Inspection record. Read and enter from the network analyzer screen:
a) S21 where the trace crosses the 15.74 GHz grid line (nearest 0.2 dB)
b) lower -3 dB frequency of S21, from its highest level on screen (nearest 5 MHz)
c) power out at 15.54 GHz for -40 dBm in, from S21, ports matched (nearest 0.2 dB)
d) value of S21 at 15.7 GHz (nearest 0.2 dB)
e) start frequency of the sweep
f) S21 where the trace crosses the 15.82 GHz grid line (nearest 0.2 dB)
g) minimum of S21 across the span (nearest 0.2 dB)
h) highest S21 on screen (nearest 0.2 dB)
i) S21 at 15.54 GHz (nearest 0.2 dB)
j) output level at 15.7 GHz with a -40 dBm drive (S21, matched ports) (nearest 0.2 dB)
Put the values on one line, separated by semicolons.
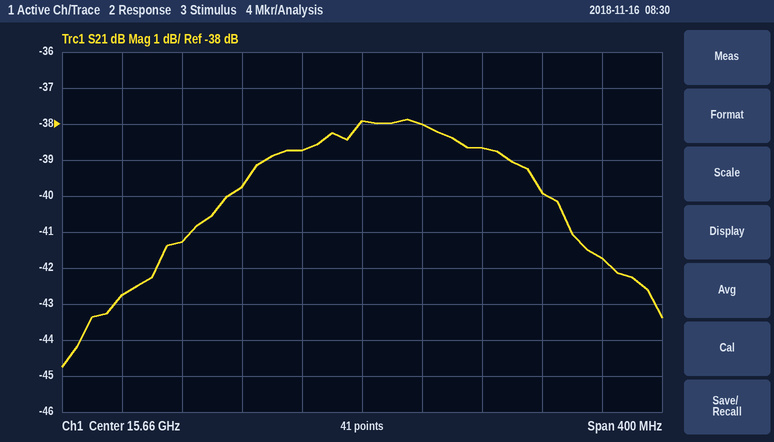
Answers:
-38.6 dB; 15.550 GHz; -81.2 dBm; -38.0 dB; 15.46 GHz; -41.8 dB; -44.8 dB; -37.8 dB; -41.2 dB; -78.0 dBm
